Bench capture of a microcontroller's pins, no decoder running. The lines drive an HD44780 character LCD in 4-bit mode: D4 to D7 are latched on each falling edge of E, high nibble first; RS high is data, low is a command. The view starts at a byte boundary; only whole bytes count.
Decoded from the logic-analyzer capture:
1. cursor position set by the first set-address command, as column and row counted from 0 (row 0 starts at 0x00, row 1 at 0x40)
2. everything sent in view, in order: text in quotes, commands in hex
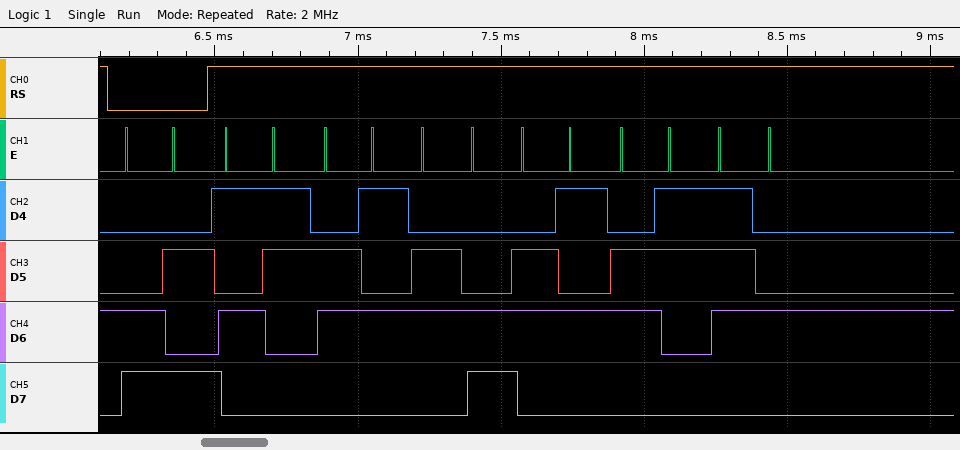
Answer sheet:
column 10, row 1
0xCA "Select"
